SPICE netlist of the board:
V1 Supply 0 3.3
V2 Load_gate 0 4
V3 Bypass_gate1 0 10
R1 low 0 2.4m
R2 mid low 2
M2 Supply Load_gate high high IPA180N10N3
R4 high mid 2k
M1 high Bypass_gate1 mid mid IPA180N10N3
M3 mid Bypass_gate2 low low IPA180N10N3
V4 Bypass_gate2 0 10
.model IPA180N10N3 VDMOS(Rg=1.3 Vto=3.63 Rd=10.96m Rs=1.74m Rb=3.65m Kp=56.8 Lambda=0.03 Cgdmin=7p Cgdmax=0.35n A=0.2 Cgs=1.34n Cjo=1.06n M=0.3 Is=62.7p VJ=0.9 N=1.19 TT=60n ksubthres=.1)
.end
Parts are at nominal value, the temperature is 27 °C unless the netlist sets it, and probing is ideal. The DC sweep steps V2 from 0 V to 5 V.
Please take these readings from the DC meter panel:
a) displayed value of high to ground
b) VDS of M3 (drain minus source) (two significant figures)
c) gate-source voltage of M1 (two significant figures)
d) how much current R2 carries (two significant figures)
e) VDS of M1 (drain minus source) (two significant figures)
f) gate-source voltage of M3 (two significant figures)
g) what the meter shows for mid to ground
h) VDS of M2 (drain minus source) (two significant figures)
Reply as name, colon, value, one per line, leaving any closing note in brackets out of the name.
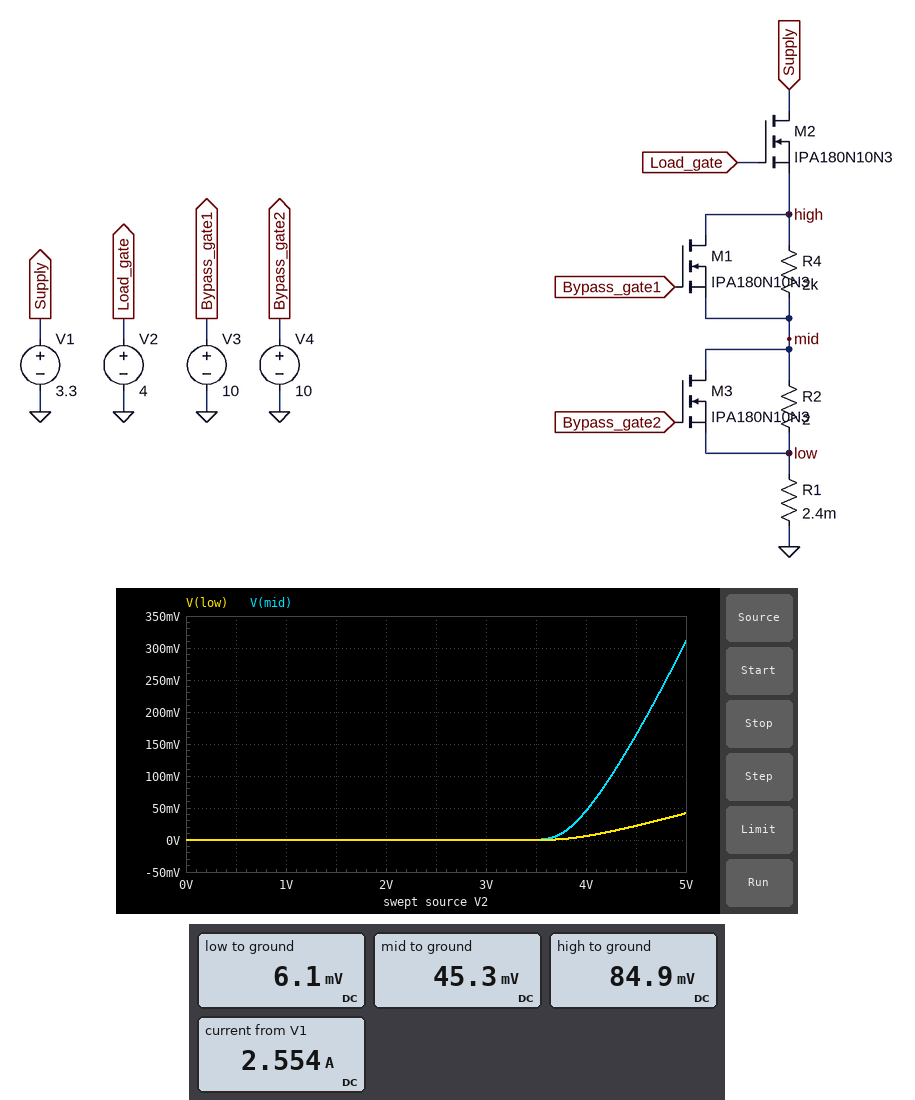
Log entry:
displayed value of high to ground: 84.9 mV
VDS of M3 (drain minus source): 39 mV
gate-source voltage of M1: 10 V
how much current R2 carries: 20 mA
VDS of M1 (drain minus source): 40 mV
gate-source voltage of M3: 10 V
what the meter shows for mid to ground: 45.3 mV
VDS of M2 (drain minus source): 3.2 V
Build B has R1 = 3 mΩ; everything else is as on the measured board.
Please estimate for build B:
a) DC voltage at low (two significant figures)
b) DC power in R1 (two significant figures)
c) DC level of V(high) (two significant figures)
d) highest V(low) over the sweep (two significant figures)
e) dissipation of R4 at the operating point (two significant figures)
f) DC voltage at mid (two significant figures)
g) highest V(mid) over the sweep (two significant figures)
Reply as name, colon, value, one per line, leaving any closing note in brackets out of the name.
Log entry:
DC voltage at low: 7.6 mV
DC power in R1: 19 mW
DC level of V(high): 86 mV
highest V(low) over the sweep: 52 mV
dissipation of R4 at the operating point: 770 nW
DC voltage at mid: 47 mV
highest V(mid) over the sweep: 320 mV
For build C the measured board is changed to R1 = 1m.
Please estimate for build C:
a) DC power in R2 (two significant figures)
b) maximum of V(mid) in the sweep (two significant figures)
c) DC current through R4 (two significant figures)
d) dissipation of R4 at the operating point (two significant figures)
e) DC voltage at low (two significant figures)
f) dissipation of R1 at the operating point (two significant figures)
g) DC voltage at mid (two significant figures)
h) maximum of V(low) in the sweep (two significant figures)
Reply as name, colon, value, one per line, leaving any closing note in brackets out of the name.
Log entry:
DC power in R2: 790 µW
maximum of V(mid) in the sweep: 290 mV
DC current through R4: 20 µA
dissipation of R4 at the operating point: 810 nW
DC voltage at low: 2.6 mV
dissipation of R1 at the operating point: 6.7 mW
DC voltage at mid: 42 mV
maximum of V(low) in the sweep: 18 mV
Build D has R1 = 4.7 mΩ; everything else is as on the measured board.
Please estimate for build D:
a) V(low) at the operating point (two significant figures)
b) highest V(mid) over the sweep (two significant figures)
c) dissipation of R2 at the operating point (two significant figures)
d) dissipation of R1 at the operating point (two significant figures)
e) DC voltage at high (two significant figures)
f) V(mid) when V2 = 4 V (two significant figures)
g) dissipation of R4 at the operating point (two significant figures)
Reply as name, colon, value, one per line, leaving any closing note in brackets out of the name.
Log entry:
V(low) at the operating point: 12 mV
highest V(mid) over the sweep: 340 mV
dissipation of R2 at the operating point: 730 µW
dissipation of R1 at the operating point: 29 mW
DC voltage at high: 89 mV
V(mid) when V2 = 4 V: 50 mV
dissipation of R4 at the operating point: 750 nW
